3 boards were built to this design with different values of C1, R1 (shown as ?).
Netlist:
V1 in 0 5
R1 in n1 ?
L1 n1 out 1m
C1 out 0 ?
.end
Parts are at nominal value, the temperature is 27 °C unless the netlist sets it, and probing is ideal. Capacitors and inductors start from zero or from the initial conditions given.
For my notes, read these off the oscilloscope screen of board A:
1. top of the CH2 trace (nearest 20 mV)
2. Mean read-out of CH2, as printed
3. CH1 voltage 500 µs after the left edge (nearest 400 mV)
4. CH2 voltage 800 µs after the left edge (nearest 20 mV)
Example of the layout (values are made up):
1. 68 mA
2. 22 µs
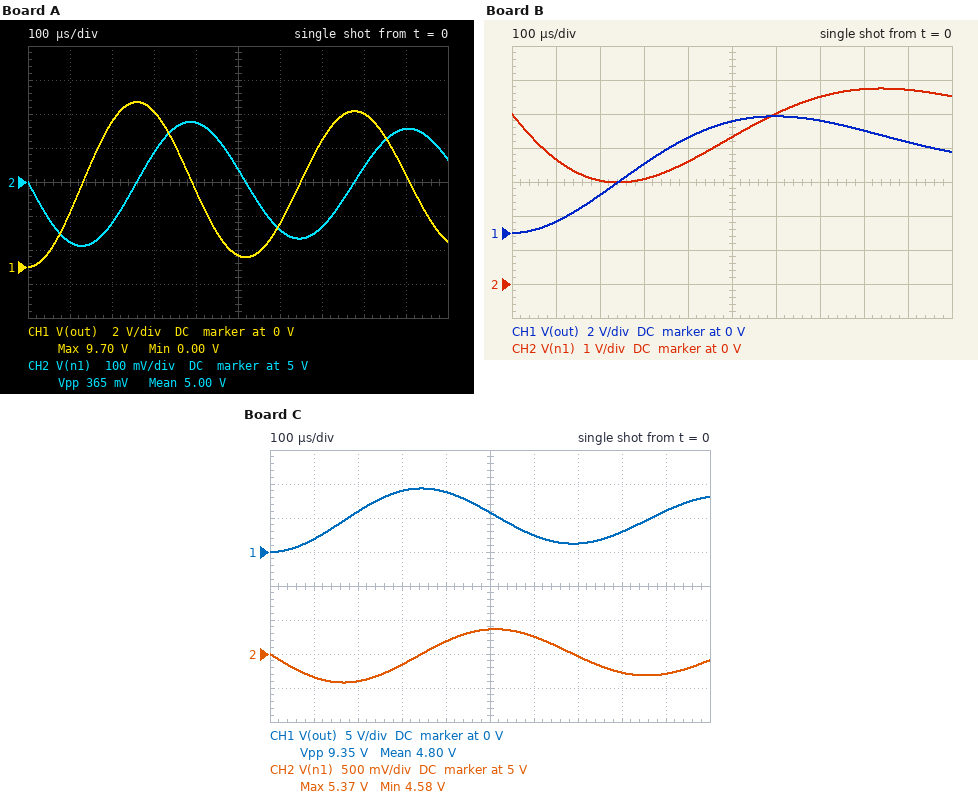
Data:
1. 5.18 V
2. 5.00 V
3. 800 mV
4. 5.04 V
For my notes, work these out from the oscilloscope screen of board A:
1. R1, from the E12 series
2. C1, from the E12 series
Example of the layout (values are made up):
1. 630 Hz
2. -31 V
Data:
1. 0.47 Ω
2. 6.8 µF
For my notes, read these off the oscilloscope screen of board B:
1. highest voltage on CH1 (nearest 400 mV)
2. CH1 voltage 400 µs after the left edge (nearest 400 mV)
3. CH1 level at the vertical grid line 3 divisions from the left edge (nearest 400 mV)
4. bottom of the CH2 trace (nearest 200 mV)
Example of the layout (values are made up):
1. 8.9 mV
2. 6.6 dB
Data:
1. 6.8 V
2. 5.6 V
3. 4.0 V
4. 3.0 V
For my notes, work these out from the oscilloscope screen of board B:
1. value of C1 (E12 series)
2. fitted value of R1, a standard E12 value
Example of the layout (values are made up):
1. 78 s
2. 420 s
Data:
1. 33 µF
2. 3.3 Ω
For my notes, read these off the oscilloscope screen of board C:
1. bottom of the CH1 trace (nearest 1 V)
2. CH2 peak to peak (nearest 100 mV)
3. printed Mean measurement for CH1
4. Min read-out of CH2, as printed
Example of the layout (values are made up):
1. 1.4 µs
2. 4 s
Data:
1. 0 V
2. 800 mV
3. 4.80 V
4. 4.58 V
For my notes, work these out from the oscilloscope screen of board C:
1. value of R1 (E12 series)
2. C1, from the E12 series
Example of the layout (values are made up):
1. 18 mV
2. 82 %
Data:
1. 0.82 Ω
2. 12 µF
